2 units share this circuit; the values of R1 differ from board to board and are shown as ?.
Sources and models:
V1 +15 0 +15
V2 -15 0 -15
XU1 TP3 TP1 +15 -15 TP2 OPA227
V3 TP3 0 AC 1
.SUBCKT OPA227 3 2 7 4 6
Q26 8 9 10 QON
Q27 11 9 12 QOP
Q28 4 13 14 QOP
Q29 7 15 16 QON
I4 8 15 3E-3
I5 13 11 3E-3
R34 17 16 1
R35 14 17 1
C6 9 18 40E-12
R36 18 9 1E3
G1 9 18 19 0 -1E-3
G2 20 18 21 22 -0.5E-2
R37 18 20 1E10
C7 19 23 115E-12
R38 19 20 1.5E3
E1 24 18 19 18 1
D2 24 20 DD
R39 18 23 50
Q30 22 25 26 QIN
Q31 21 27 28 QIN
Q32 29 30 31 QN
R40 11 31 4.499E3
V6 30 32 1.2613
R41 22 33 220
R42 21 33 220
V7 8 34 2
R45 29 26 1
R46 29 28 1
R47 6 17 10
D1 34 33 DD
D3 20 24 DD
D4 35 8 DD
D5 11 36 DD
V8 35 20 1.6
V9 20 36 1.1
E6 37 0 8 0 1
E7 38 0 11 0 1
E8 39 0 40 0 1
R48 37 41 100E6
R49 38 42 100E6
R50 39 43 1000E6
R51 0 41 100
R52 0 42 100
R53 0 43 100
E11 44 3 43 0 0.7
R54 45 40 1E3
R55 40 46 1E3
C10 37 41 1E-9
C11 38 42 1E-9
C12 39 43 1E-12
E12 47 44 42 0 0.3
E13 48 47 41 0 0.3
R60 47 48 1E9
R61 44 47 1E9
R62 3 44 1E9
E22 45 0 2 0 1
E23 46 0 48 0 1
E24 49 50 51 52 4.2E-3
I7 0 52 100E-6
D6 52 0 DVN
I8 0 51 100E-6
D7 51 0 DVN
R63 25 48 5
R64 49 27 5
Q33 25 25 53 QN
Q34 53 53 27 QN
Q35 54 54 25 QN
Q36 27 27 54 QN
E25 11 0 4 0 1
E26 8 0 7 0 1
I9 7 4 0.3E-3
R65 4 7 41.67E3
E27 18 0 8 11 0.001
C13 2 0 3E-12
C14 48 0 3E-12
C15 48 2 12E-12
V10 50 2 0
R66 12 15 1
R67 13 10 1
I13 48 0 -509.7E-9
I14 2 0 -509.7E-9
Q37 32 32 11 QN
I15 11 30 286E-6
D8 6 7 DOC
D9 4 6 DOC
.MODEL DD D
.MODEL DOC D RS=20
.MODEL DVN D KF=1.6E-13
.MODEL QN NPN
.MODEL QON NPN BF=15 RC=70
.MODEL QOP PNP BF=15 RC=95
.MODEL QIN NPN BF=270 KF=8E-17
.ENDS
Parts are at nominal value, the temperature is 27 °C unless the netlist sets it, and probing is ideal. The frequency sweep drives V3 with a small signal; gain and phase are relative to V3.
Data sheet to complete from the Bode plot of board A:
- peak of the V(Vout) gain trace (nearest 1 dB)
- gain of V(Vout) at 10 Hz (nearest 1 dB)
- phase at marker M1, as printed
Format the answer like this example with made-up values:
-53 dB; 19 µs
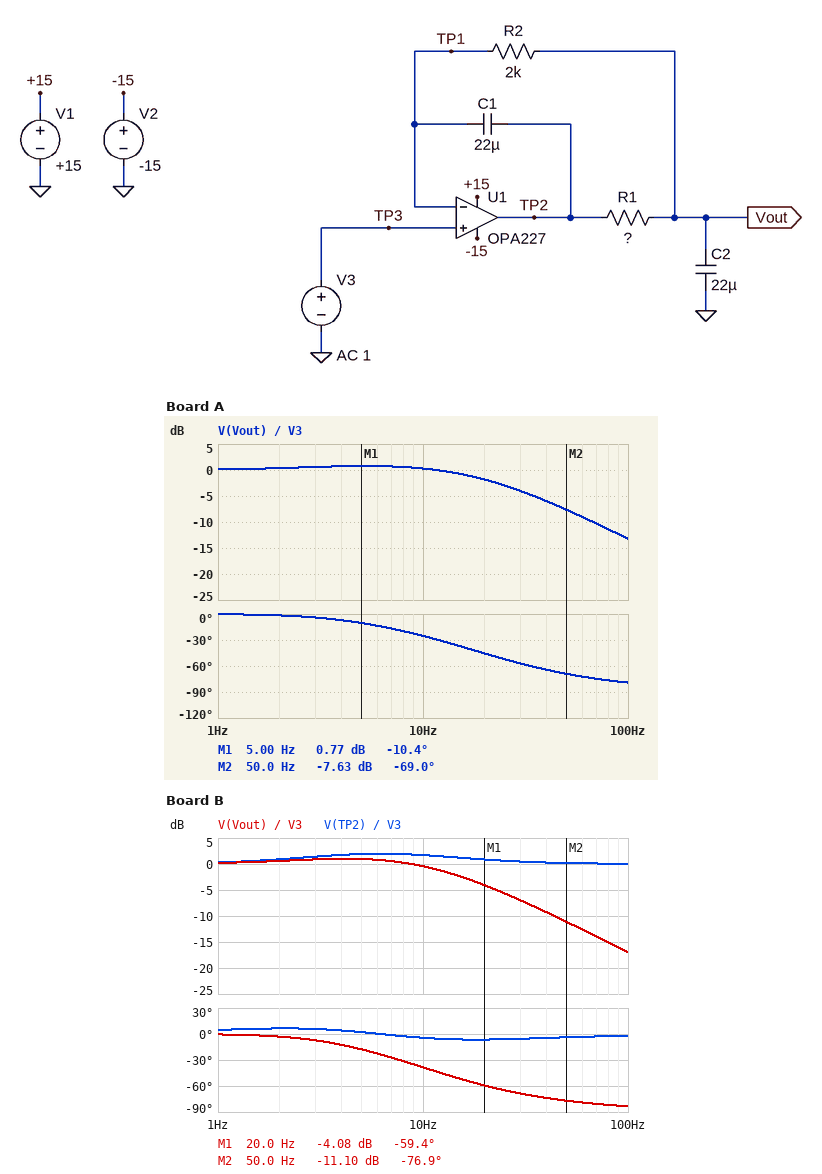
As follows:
1 dB; 0 dB; -10.4 deg
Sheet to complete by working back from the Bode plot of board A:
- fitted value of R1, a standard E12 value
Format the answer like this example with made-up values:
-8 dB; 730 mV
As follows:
390 Ω
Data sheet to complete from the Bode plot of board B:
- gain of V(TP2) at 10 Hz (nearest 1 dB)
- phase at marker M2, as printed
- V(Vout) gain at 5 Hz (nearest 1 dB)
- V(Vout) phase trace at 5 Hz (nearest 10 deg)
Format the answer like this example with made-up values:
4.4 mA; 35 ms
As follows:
2 dB; -76.9 deg; 1 dB; -20 deg
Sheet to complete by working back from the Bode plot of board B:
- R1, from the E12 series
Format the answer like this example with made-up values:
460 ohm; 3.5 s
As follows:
680 Ω
